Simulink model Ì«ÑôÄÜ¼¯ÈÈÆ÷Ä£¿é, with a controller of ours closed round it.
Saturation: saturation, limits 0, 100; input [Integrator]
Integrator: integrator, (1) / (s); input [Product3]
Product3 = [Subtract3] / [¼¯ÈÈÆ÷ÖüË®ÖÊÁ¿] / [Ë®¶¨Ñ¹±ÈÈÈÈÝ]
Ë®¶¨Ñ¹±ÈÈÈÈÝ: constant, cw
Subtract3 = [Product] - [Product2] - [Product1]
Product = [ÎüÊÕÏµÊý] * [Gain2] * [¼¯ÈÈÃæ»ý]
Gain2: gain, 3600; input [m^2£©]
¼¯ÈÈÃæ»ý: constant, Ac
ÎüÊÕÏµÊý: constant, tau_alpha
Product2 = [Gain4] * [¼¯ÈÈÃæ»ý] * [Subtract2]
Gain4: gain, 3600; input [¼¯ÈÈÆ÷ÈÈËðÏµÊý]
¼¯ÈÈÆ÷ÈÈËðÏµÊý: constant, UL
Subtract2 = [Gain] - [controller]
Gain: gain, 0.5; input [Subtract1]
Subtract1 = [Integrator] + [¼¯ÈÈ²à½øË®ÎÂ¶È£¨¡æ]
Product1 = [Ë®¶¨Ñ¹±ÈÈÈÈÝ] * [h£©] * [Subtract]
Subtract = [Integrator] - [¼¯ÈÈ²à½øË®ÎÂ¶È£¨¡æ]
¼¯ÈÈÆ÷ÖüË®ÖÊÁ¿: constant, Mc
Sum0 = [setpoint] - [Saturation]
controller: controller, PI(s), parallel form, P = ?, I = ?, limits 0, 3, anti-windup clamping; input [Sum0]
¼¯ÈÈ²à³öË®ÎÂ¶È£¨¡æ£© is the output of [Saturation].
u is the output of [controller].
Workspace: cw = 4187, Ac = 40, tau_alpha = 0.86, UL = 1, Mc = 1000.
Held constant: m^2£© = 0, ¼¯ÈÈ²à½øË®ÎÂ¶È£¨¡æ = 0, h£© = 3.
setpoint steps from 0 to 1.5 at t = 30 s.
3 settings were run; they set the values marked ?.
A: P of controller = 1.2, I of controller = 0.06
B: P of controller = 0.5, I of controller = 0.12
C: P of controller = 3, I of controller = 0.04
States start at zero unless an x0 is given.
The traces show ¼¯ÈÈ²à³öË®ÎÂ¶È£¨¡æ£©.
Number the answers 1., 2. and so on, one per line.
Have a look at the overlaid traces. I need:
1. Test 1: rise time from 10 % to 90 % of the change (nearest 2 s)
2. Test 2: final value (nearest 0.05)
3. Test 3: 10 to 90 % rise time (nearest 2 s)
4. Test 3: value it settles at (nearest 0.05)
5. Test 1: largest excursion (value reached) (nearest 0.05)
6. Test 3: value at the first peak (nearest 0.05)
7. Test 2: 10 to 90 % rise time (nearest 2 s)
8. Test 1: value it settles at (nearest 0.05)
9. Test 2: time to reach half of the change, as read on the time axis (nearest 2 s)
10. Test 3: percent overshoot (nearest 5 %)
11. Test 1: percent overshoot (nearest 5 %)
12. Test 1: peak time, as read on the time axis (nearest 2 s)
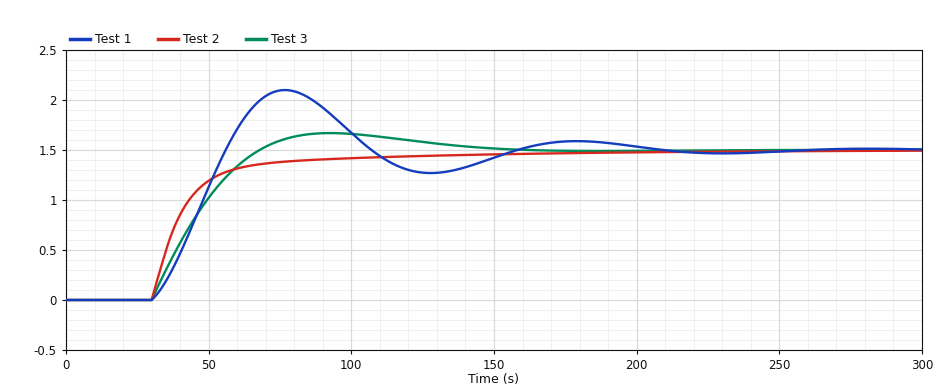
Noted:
1. 20 s
2. 1.50
3. 28 s
4. 1.50
5. 2.10
6. 1.65
7. 34 s
8. 1.50
9. 38 s
10. 10 %
11. 40 %
12. 76 s
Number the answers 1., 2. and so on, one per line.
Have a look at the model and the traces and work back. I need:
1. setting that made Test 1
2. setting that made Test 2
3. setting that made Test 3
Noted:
1. B
2. C
3. A
